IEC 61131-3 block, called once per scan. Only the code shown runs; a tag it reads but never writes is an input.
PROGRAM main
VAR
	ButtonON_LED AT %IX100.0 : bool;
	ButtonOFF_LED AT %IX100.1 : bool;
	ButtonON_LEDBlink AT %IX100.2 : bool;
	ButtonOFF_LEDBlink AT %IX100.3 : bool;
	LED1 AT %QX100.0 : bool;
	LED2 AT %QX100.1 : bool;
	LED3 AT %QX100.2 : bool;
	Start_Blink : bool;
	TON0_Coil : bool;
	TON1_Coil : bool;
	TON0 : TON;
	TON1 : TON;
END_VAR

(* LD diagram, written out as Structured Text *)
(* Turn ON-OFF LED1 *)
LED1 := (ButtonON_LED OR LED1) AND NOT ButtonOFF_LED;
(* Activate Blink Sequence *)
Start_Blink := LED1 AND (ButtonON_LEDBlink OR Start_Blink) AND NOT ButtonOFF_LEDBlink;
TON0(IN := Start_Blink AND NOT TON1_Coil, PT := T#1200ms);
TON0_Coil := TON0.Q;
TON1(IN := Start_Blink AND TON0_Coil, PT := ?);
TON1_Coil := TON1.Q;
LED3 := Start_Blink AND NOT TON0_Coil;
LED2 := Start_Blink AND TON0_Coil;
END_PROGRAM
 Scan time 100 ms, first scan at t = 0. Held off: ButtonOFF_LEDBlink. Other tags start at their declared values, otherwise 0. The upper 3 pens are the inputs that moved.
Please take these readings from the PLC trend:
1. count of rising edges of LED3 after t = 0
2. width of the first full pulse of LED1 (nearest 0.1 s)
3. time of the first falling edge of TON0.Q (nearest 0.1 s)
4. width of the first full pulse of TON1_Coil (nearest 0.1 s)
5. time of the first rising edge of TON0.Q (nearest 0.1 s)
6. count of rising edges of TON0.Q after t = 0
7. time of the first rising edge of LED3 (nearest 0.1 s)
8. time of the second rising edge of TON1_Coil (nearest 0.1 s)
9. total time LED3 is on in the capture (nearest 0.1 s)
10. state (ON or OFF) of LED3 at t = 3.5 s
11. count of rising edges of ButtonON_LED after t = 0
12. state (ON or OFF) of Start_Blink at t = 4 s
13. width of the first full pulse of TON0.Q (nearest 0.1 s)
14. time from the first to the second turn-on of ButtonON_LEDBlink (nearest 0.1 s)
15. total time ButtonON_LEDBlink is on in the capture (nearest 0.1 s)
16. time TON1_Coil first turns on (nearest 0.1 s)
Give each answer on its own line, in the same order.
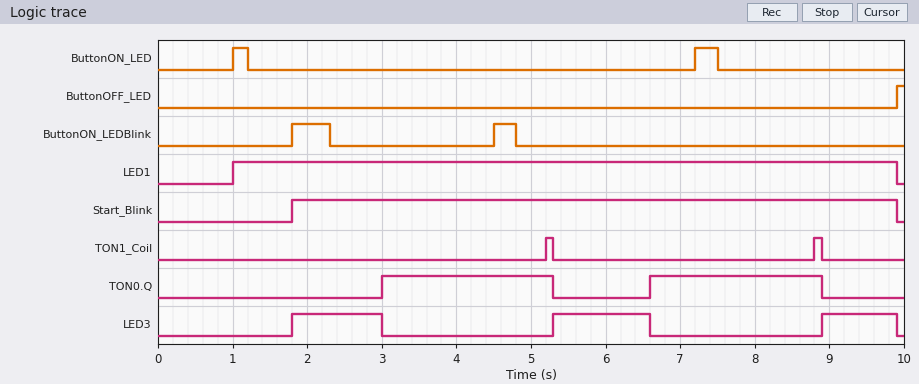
3
8.9 s
5.3 s
0.1 s
3.0 s
2
1.8 s
8.8 s
3.5 s
OFF
2
ON
2.3 s
2.7 s
0.8 s
5.2 s
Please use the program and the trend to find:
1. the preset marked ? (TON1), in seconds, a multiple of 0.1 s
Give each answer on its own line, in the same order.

2.2 s
